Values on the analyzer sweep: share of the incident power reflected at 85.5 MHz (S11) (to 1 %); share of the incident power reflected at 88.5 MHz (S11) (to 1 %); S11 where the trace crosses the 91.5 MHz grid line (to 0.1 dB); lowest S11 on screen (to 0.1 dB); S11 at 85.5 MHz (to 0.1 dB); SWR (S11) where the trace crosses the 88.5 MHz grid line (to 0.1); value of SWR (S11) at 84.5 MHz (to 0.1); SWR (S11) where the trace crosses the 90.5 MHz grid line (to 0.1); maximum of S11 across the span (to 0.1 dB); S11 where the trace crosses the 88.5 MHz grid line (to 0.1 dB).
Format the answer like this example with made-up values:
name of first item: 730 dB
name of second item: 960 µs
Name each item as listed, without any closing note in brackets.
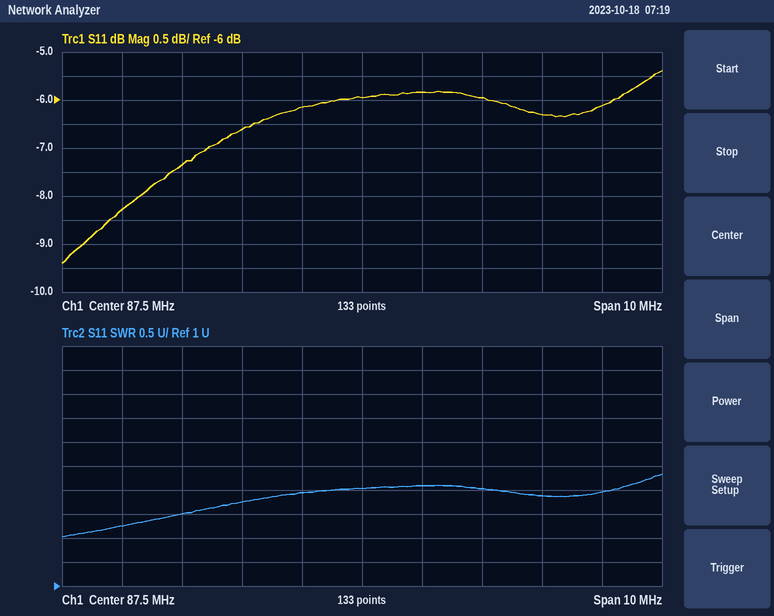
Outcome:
share of the incident power reflected at 85.5 MHz (S11): 22 %
share of the incident power reflected at 88.5 MHz (S11): 26 %
S11 where the trace crosses the 91.5 MHz grid line: -6.1 dB
lowest S11 on screen: -9.4 dB
S11 at 85.5 MHz: -6.6 dB
SWR (S11) where the trace crosses the 88.5 MHz grid line: 3.1
value of SWR (S11) at 84.5 MHz: 2.5
SWR (S11) where the trace crosses the 90.5 MHz grid line: 2.9
maximum of S11 across the span: -5.4 dB
S11 where the trace crosses the 88.5 MHz grid line: -5.8 dB
